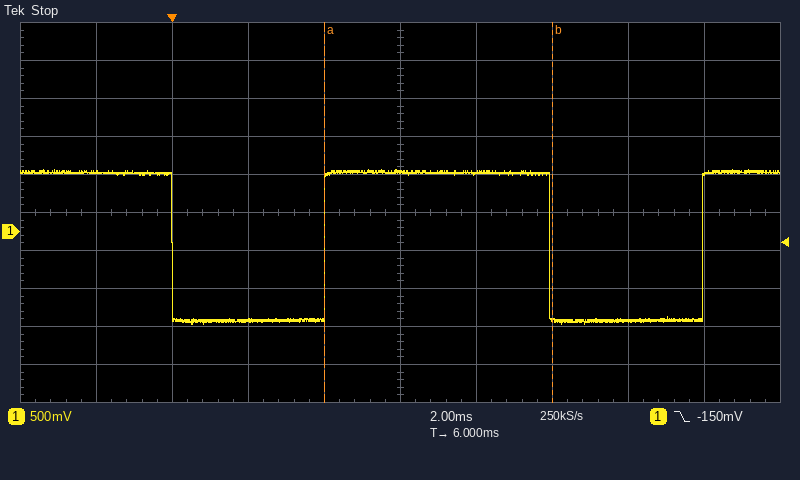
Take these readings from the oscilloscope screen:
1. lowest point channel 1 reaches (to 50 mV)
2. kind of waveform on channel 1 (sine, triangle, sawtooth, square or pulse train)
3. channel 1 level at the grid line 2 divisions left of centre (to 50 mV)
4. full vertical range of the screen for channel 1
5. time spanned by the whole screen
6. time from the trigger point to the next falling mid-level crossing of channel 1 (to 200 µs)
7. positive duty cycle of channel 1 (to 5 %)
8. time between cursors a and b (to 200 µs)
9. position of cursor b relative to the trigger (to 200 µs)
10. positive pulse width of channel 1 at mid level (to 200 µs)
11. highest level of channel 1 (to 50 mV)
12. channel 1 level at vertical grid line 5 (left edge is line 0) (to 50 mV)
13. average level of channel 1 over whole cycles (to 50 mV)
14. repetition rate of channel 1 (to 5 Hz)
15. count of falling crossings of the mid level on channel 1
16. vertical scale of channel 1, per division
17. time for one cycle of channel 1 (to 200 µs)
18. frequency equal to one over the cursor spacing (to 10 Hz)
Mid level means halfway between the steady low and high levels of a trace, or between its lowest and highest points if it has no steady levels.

-1.20 V
pulse train
-1.15 V
5 V
20 ms
10.0 ms
60 %
6.0 ms
+10.0 ms
6.0 ms
800 mV
800 mV
0 mV
100 Hz
2
500 mV
10.0 ms
170 Hz
